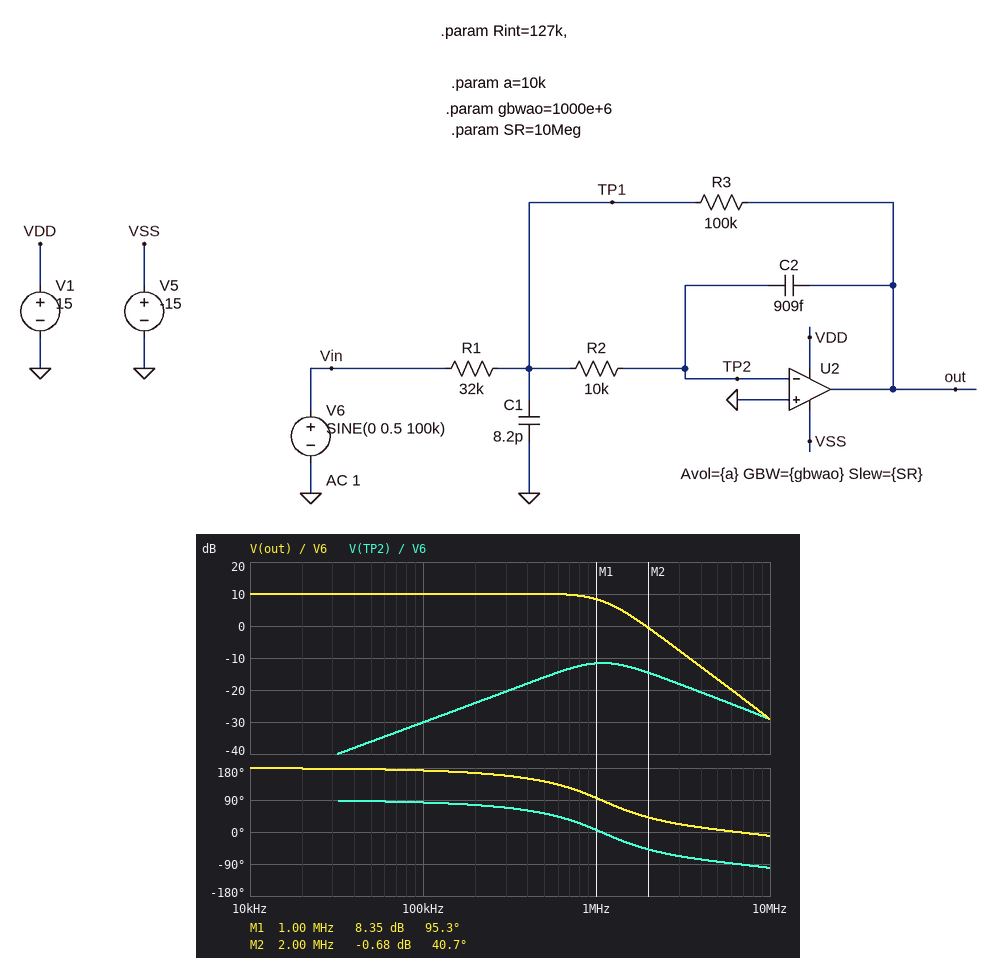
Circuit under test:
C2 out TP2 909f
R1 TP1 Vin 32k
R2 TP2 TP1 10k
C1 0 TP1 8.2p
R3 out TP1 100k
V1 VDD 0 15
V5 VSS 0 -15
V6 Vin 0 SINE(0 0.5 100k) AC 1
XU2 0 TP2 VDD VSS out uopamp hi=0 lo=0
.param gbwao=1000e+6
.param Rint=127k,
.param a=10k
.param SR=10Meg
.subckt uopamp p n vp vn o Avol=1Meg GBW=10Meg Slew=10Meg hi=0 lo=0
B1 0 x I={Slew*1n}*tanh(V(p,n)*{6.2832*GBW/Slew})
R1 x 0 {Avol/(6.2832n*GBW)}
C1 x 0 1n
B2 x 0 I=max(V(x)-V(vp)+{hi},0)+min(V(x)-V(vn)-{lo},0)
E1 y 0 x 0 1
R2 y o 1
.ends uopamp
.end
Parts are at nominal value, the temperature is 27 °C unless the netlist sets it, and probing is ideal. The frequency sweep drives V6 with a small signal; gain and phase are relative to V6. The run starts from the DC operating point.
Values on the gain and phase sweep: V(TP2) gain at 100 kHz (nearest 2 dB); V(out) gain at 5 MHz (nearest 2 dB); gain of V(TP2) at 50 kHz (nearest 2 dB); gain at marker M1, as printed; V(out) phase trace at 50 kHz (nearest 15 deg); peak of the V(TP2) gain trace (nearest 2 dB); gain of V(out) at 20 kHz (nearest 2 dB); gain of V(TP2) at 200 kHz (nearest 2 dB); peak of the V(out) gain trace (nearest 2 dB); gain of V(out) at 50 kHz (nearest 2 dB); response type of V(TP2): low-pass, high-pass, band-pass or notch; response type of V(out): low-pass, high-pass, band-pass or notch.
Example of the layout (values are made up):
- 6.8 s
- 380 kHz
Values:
- -30 dB
- -16 dB
- -36 dB
- 8.35 dB
- 180 deg
- -12 dB
- 10 dB
- -24 dB
- 10 dB
- 10 dB
- band-pass
- low-pass
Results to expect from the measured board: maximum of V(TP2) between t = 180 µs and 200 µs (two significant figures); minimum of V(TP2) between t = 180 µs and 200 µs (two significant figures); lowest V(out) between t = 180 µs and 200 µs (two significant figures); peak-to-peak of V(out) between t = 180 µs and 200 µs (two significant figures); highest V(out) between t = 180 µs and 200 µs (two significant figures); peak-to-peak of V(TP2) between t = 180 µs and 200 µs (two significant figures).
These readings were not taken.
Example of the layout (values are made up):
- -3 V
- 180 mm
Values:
- 16 mV
- -16 mV
- -1.6 V
- 3.1 V
- 1.6 V
- 31 mV
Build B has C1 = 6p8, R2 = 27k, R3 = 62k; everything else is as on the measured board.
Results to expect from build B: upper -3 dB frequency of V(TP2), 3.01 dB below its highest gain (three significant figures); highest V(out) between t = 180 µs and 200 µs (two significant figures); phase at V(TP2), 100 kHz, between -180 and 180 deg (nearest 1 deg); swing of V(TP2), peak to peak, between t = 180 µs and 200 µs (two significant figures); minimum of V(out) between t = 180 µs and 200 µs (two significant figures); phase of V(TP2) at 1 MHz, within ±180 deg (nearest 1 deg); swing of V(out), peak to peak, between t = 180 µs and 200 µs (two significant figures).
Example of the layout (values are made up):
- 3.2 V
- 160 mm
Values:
- 2.16 MHz
- 970 mV
- 84 deg
- 19 mV
- -970 mV
- 13 deg
- 1.9 V
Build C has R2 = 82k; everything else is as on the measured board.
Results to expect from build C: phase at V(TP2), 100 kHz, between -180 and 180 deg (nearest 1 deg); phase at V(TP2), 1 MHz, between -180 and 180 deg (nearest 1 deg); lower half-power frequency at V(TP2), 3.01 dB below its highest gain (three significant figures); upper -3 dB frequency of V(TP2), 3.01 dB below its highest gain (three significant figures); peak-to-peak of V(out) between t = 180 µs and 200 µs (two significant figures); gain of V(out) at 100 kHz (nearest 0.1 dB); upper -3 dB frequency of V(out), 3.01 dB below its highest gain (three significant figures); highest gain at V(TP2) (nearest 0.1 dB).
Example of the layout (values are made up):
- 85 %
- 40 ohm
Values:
- 73 deg
- -39 deg
- 274 kHz
- 1.23 MHz
- 3.1 V
- 9.8 dB
- 487 kHz
- -19.2 dB
